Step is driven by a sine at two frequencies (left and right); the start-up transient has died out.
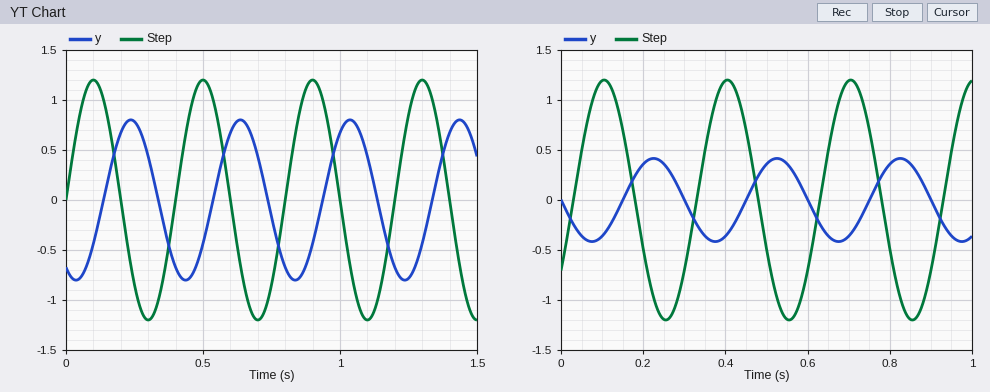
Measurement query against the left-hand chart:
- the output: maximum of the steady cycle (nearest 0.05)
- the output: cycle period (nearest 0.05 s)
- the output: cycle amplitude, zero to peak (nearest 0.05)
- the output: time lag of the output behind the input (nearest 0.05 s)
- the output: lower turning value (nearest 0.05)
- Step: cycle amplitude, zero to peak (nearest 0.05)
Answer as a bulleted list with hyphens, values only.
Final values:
- 0.80
- 0.40 s
- 0.80
- 0.15 s
- -0.80
- 1.20
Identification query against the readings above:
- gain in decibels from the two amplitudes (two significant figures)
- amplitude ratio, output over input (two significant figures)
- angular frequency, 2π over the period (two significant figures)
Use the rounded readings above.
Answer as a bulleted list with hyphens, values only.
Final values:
- -3.5 dB
- 0.67
- 16 rad/s
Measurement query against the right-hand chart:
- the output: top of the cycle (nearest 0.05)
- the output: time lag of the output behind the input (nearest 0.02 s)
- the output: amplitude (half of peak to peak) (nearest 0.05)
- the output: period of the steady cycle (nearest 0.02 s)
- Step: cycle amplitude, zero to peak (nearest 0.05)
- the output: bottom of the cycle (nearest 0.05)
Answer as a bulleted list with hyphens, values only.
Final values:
- 0.40
- 0.12 s
- 0.40
- 0.30 s
- 1.20
- -0.40
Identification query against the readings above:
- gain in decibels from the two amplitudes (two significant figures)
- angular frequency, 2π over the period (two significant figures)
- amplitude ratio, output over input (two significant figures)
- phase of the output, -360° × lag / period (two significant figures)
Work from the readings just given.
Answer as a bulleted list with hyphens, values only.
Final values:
- -9.5 dB
- 21 rad/s
- 0.33
- -140°
